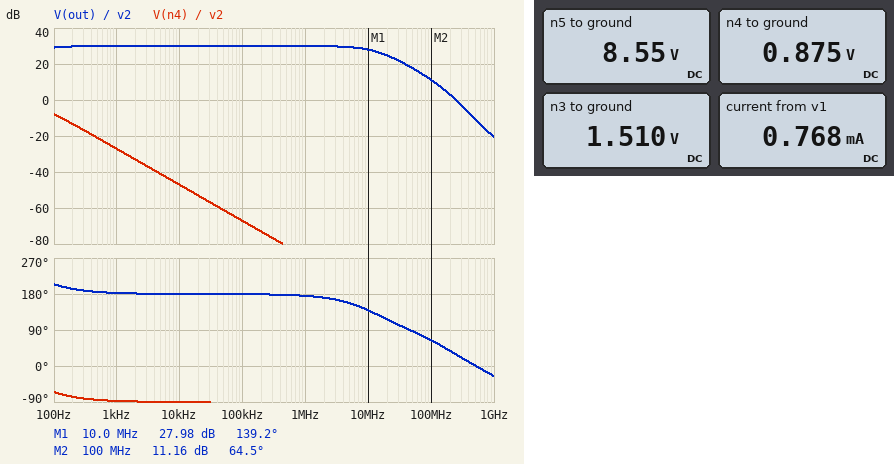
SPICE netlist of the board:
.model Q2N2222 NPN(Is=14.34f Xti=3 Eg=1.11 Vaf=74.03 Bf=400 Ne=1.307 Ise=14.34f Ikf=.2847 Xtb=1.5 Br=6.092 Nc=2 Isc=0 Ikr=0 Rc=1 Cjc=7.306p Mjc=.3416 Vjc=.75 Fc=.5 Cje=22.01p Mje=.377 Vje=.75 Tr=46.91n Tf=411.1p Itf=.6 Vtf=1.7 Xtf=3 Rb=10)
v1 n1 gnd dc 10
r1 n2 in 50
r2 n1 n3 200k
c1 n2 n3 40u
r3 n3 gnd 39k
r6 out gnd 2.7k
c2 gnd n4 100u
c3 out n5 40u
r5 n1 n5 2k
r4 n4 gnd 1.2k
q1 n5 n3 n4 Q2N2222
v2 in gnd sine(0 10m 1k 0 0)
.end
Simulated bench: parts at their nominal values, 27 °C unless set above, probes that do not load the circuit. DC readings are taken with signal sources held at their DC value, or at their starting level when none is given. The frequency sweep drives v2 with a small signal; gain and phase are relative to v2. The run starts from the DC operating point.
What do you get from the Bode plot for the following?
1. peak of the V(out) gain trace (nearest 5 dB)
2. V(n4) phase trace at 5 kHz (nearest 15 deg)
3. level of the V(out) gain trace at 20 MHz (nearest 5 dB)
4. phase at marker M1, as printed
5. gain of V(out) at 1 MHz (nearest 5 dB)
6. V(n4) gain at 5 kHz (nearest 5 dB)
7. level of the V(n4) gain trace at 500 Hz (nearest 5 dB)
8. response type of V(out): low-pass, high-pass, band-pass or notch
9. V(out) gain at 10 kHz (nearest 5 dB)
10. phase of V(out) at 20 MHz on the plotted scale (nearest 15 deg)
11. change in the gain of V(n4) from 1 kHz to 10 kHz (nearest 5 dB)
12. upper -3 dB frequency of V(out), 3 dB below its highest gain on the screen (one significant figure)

30 dB
-90 deg
25 dB
139.2 deg
30 dB
-40 dB
-20 dB
low-pass
30 dB
120 deg
-20 dB
10 MHz
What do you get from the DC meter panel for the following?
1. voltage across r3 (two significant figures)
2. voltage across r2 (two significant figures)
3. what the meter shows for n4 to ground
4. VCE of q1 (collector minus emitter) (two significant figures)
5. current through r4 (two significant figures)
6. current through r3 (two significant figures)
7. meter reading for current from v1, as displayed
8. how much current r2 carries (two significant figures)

1.5 V
8.5 V
0.875 V
7.7 V
730 µA
39 µA
0.768 mA
42 µA
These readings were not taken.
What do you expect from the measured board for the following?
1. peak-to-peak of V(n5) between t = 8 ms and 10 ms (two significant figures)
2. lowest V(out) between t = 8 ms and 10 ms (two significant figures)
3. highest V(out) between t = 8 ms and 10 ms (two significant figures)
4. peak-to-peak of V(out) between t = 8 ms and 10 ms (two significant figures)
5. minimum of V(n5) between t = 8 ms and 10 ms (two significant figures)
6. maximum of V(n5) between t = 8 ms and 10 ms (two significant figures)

620 mV
-340 mV
280 mV
620 mV
8.2 V
8.8 V
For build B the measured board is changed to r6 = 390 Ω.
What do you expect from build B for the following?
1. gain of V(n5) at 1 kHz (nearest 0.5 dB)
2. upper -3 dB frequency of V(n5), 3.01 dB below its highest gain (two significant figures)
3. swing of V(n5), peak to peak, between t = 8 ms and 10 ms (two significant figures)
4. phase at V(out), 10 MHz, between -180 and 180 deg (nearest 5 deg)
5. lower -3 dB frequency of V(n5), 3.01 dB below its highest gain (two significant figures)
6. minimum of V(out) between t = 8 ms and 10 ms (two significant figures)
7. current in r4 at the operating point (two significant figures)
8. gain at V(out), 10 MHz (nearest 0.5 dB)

19.0 dB
30 MHz
180 mV
160 deg
44 Hz
-98 mV
730 µA
18.5 dB
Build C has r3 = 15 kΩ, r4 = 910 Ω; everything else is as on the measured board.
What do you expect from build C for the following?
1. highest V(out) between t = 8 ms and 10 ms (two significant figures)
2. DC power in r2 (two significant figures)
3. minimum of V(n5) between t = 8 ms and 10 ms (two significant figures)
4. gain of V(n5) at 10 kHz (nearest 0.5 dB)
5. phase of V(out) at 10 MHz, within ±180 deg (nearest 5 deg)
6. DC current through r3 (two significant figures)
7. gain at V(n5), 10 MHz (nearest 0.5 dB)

42 mV
430 µW
9.7 V
14.0 dB
155 deg
46 µA
13.5 dB
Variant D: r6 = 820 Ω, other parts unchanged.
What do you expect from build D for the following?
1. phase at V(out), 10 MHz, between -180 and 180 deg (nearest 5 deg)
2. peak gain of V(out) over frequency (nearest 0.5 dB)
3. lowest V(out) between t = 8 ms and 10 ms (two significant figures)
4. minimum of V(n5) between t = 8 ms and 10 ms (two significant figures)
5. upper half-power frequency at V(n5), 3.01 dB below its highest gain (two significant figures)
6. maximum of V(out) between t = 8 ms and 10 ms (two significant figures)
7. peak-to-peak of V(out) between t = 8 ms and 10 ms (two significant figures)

150 deg
24.0 dB
-170 mV
8.4 V
21 MHz
140 mV
320 mV
